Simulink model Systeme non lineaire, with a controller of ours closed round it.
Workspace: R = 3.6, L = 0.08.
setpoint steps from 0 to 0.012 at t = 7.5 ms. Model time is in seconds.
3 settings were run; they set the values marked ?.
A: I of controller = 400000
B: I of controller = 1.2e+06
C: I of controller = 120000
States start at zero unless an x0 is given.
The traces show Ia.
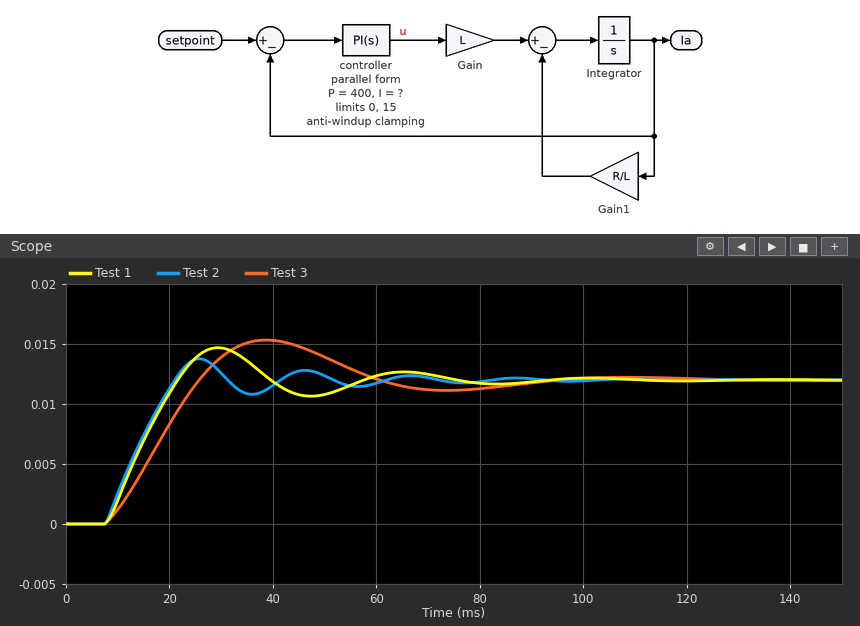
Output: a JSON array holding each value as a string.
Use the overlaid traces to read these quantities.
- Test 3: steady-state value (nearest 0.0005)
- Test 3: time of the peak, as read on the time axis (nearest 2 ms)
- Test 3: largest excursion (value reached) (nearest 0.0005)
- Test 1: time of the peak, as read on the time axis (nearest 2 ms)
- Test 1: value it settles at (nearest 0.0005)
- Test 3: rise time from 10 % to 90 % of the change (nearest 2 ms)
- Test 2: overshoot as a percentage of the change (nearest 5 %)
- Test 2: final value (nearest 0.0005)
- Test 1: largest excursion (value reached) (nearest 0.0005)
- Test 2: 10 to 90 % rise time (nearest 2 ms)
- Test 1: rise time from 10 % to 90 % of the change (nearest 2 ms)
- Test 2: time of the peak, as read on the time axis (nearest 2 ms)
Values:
["0.0120", "38 ms", "0.0155", "30 ms", "0.0120", "14 ms", "15 %", "0.0120", "0.0145", "10 ms", "10 ms", "26 ms"]
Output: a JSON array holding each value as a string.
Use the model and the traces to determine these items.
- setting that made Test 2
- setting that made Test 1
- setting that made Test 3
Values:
["B", "A", "C"]
